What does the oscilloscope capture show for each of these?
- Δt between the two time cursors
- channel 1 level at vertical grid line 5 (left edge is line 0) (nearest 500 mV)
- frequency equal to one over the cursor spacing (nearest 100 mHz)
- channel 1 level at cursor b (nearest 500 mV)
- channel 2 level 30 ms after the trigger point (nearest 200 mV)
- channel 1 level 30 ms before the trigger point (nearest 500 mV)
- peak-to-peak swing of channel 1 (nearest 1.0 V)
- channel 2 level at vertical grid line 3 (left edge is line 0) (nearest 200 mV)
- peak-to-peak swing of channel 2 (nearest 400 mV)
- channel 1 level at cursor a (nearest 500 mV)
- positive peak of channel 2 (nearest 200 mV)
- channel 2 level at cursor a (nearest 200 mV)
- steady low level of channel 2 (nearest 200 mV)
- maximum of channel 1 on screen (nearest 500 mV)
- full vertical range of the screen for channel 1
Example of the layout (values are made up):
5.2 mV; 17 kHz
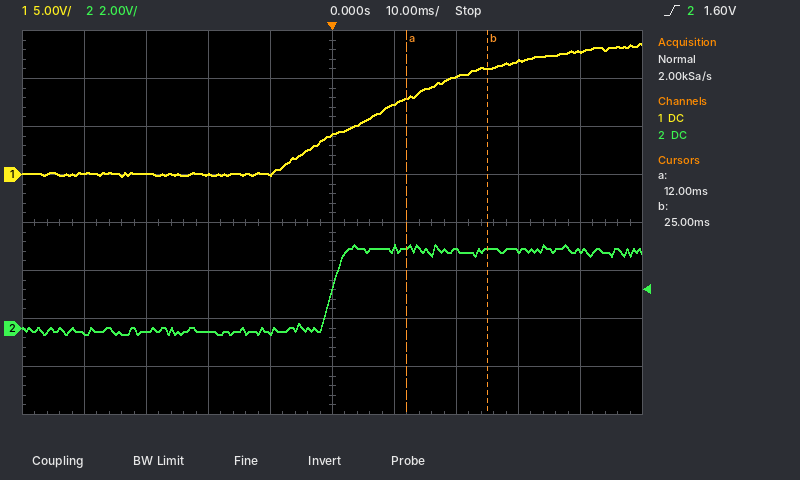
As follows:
13 ms; 4.0 V; 76.9 Hz; 11.0 V; 3.2 V; 0.0 V; 14.0 V; -200 mV; 3.6 V; 8.0 V; 3.4 V; 3.4 V; -200 mV; 13.5 V; 40 V
